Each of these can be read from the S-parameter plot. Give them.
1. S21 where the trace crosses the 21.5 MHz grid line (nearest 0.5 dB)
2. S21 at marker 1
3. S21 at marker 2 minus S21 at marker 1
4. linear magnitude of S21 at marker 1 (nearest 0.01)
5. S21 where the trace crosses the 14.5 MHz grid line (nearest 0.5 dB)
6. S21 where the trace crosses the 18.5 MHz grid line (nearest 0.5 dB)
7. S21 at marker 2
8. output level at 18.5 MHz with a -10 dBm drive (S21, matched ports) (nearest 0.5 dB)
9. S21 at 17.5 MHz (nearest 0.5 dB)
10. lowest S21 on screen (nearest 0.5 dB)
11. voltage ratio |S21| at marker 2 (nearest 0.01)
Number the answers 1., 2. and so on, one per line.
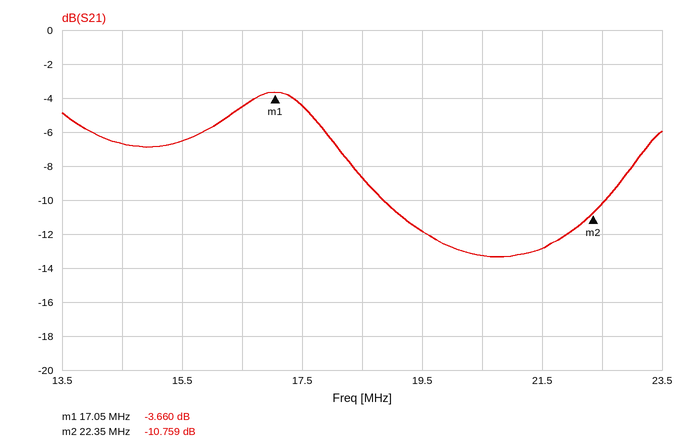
1. -13.0 dB
2. -3.660 dB
3. -7.099 dB
4. 0.66
5. -6.5 dB
6. -8.5 dB
7. -10.759 dB
8. -18.5 dBm
9. -4.5 dB
10. -13.5 dB
11. 0.29
